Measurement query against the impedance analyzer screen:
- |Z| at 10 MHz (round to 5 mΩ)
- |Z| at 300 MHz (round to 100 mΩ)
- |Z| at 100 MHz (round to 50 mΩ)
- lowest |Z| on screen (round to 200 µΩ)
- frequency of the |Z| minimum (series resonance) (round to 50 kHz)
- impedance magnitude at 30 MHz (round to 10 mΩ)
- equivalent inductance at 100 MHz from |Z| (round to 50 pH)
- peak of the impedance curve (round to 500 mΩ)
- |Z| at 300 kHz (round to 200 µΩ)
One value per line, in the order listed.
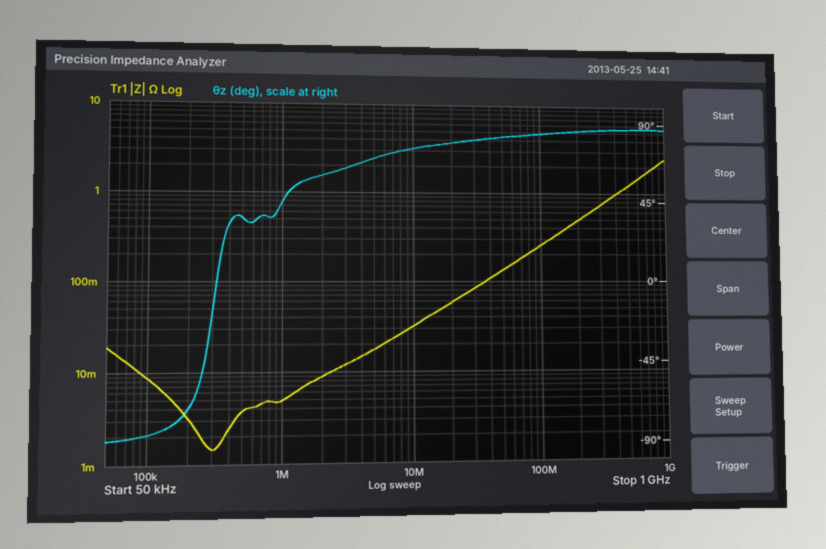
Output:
30 mΩ
700 mΩ
250 mΩ
1.4 mΩ
300 kHz
80 mΩ
400 pH
2.5 Ω
1.4 mΩ
